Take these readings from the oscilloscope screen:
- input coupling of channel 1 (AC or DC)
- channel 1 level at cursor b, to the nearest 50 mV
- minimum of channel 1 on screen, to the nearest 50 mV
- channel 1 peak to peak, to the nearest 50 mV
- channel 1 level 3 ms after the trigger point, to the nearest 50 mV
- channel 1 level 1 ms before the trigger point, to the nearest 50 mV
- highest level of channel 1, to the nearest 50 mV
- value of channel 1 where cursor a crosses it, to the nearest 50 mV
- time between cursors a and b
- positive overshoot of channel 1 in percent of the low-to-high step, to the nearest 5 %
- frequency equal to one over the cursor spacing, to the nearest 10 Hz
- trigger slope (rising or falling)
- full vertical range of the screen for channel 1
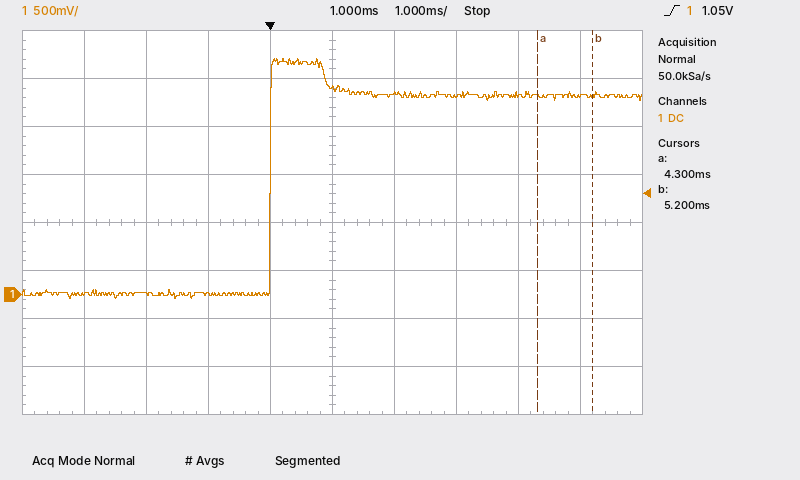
DC
2.10 V
-50 mV
2.50 V
2.05 V
0 mV
2.45 V
2.05 V
900 µs
20 %
1.11 kHz
rising
4 V
